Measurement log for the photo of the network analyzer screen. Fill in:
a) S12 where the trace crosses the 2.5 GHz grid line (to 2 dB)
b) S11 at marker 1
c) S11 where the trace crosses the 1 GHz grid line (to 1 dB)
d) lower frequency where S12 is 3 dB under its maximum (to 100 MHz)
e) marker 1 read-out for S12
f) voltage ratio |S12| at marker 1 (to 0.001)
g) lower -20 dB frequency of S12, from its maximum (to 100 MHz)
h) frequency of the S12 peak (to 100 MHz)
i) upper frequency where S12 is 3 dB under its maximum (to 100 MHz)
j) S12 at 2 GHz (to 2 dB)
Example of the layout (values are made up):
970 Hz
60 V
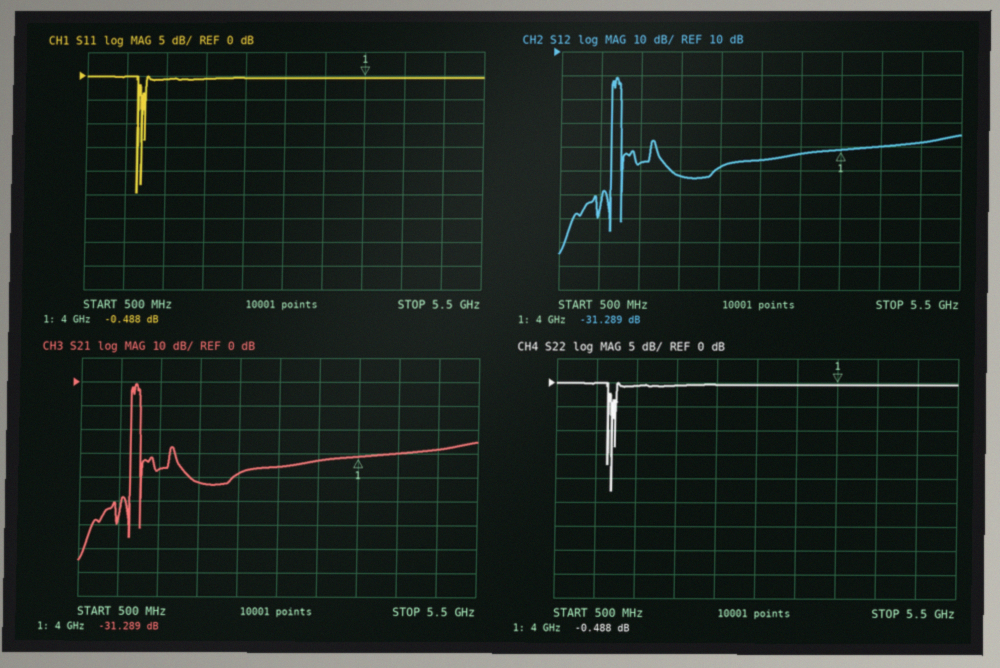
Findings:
-38 dB
-0.488 dB
0 dB
1.2 GHz
-31.289 dB
0.027
1.1 GHz
1.2 GHz
1.2 GHz
-42 dB
